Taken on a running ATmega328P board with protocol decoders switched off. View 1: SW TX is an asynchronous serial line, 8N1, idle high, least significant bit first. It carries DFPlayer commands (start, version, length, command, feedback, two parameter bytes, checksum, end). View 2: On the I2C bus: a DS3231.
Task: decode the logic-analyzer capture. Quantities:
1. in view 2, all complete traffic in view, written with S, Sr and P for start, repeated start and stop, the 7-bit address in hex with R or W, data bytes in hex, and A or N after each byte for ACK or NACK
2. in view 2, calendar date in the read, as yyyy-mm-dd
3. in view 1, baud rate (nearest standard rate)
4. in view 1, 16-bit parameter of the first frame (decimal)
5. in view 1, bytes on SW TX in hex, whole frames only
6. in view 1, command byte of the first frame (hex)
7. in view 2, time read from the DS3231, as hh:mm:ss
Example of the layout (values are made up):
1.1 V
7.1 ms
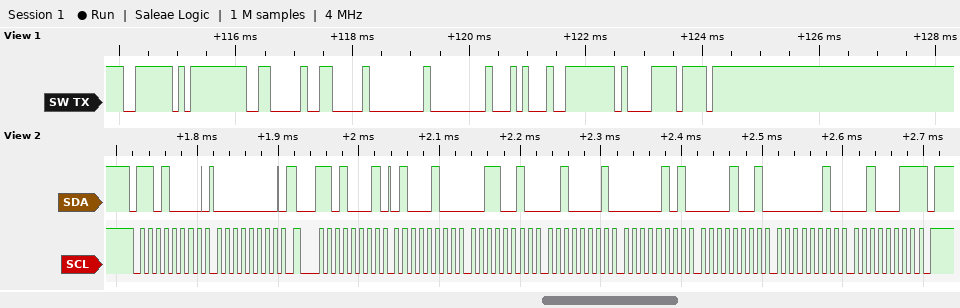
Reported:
S 68W A 00 A Sr 68R A 44 A 32 A 21 A 05 A 09 A 02 A 23 N P
2023-02-09
9600 baud
20
7E FF 06 06 00 00 14 FE E1 EF
0x06
21:32:44
